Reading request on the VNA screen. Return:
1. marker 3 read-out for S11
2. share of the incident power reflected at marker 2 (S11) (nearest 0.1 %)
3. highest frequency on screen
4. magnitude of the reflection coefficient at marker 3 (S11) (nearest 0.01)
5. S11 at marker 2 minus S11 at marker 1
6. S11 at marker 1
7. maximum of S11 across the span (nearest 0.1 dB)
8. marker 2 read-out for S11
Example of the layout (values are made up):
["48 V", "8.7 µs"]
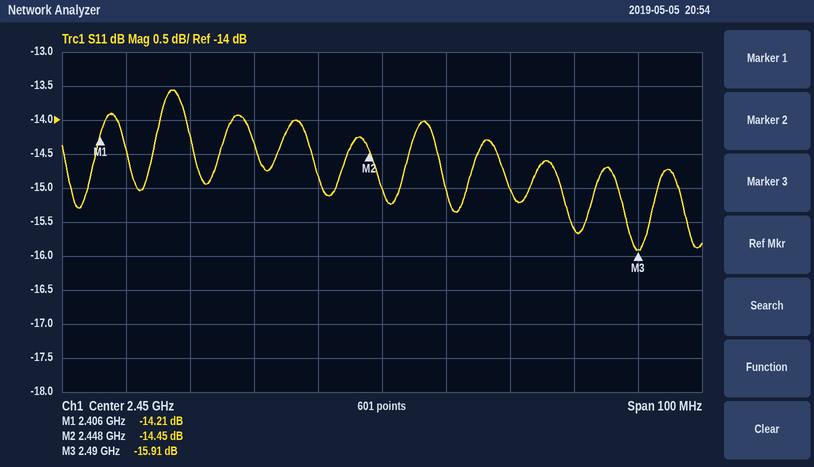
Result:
["-15.91 dB", "3.6 %", "2.5 GHz", "0.16", "-0.24 dB", "-14.21 dB", "-13.6 dB", "-14.45 dB"]
